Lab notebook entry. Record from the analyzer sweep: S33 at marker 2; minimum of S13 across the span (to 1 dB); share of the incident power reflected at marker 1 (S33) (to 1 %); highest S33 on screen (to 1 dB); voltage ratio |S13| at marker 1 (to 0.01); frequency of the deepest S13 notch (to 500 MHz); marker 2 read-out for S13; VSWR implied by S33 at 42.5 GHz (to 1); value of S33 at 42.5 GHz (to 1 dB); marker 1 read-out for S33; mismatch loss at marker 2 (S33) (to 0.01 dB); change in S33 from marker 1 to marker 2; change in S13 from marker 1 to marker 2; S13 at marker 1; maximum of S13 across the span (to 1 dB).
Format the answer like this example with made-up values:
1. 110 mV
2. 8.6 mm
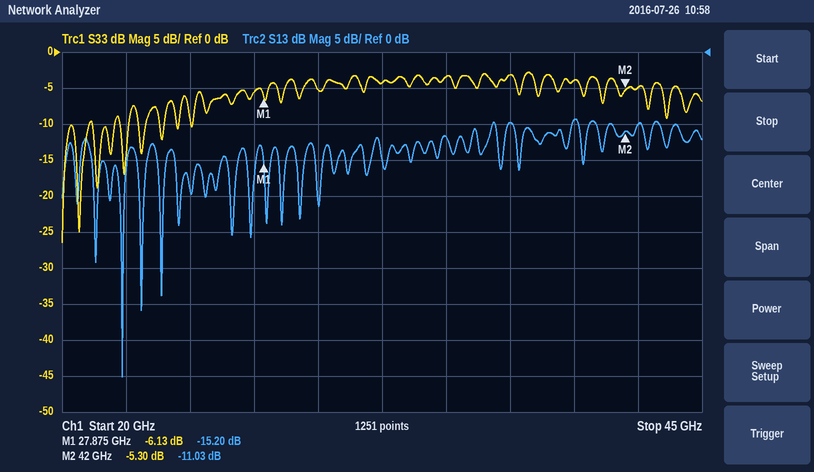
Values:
1. -5.30 dB
2. -45 dB
3. 24 %
4. -3 dB
5. 0.17
6. 22.5 GHz
7. -11.03 dB
8. 4
9. -5 dB
10. -6.13 dB
11. 1.52 dB
12. 0.83 dB
13. 4.17 dB
14. -15.20 dB
15. -9 dB
